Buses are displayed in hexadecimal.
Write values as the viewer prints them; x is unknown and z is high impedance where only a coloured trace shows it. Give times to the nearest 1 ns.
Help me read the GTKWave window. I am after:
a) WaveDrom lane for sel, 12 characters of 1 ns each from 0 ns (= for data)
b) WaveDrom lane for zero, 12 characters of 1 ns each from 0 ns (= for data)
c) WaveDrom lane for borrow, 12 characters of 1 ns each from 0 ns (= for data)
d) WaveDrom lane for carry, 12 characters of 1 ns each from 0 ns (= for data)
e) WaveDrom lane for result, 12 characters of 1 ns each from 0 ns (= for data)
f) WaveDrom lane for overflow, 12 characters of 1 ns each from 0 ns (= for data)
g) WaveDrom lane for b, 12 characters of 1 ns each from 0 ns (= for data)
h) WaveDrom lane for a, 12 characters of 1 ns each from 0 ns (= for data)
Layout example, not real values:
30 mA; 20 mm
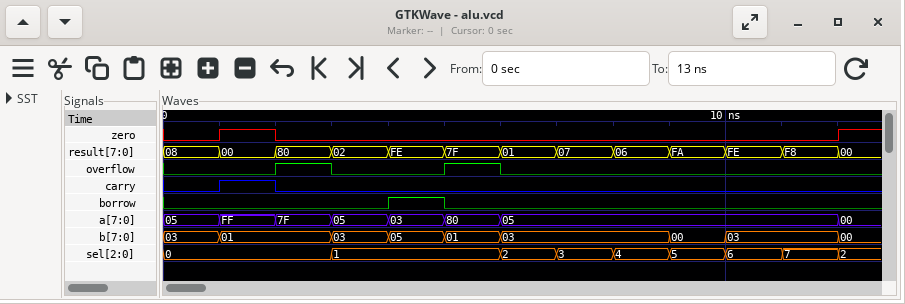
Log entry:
{name: 'sel', wave: '=..=..======', data: '0 1 2 3 4 5 6 7'}; {name: 'zero', wave: '010.........'}; {name: 'borrow', wave: '0...10......'}; {name: 'carry', wave: '010.........'}; {name: 'result', wave: '============', data: '08 00 80 02 FE 7F 01 07 06 FA FE F8'}; {name: 'overflow', wave: '0.10.10.....'}; {name: 'b', wave: '==.====..==.', data: '03 01 03 05 01 03 00 03'}; {name: 'a', wave: '=======.....', data: '05 FF 7F 05 03 80 05'}
